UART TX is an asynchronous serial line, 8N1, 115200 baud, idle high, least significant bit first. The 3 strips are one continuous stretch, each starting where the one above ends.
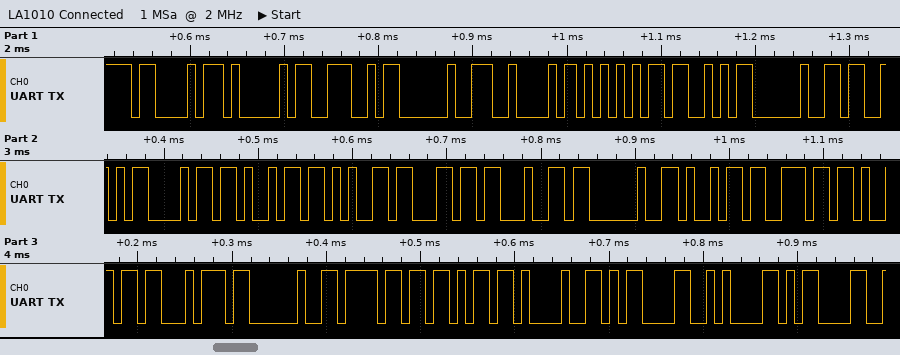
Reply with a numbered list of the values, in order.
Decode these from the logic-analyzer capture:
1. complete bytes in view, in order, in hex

1. 43 41 4E 20 42 55 53 20 53 68 69 65 6C 64 20 69 6E 69 74 20 6F 6B 21 0D 0A 0D
